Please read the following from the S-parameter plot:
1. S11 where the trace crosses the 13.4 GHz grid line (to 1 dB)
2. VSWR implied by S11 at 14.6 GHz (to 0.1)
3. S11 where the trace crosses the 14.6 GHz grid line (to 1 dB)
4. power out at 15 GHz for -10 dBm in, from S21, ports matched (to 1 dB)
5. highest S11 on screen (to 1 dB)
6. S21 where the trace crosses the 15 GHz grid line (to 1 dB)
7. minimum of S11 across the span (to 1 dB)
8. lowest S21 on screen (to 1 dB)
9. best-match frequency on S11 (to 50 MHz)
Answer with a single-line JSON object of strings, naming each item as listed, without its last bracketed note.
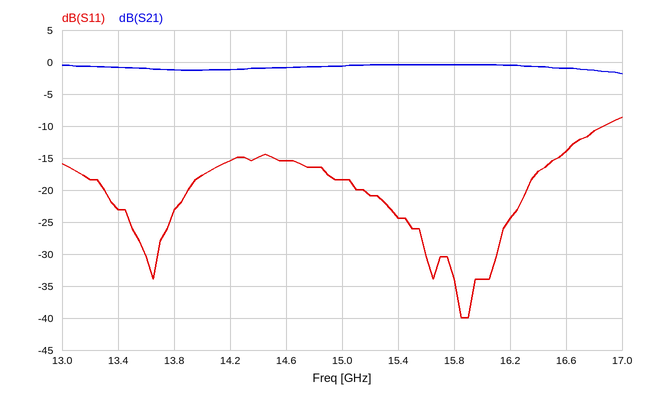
{"S11 where the trace crosses the 13.4 GHz grid line": "-23 dB", "VSWR implied by S11 at 14.6 GHz": "1.4", "S11 where the trace crosses the 14.6 GHz grid line": "-15 dB", "power out at 15 GHz for -10 dBm in, from S21, ports matched": "-11 dBm", "highest S11 on screen": "-9 dB", "S21 where the trace crosses the 15 GHz grid line": "-1 dB", "minimum of S11 across the span": "-40 dB", "lowest S21 on screen": "-2 dB", "best-match frequency on S11": "15.85 GHz"}
